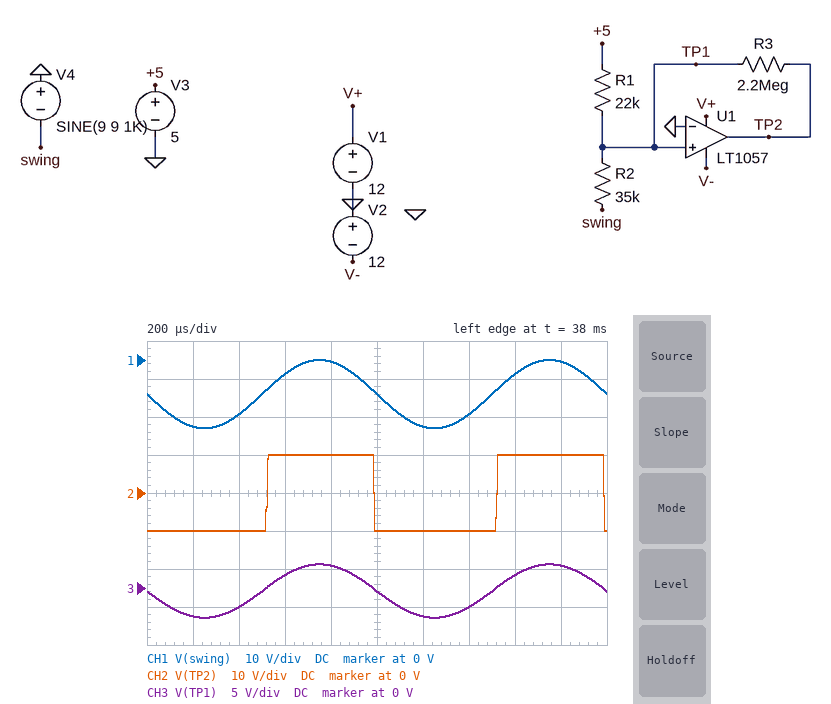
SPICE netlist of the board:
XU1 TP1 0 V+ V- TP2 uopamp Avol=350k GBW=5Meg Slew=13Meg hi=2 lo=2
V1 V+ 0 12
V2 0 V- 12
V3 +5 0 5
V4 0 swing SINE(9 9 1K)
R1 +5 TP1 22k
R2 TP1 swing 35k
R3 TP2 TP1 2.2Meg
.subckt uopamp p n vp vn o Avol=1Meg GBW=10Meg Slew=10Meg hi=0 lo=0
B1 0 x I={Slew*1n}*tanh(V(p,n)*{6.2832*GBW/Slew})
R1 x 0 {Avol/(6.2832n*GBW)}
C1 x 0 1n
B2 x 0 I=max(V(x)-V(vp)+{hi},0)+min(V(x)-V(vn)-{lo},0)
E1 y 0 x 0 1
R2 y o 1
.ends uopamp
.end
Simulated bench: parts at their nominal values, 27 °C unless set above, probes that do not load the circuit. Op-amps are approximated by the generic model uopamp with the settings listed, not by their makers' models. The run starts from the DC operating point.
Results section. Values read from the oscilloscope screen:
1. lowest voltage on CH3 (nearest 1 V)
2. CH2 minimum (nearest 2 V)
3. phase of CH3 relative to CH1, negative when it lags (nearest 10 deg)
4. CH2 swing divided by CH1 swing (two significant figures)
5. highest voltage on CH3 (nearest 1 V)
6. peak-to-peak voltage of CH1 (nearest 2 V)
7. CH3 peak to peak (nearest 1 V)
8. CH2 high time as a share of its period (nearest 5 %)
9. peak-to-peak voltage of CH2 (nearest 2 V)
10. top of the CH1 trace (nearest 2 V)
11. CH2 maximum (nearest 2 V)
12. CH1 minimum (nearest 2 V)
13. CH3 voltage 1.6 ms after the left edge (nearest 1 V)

-4 V
-10 V
0 deg
1.1
3 V
18 V
7 V
45 %
20 V
0 V
10 V
-18 V
2 V
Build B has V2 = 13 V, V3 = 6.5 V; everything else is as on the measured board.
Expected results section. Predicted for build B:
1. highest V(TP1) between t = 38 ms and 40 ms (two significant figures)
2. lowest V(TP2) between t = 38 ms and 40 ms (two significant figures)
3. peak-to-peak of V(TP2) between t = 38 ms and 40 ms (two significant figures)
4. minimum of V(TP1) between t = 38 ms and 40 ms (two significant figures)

4.0 V
-11 V
21 V
-3.0 V
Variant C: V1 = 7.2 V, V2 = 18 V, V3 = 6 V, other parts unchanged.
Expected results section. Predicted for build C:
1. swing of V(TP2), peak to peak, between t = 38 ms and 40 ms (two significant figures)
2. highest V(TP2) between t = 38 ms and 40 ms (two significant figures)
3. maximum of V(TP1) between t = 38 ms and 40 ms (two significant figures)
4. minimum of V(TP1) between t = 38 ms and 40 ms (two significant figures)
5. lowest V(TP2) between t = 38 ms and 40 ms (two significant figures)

21 V
5.2 V
3.7 V
-3.3 V
-16 V
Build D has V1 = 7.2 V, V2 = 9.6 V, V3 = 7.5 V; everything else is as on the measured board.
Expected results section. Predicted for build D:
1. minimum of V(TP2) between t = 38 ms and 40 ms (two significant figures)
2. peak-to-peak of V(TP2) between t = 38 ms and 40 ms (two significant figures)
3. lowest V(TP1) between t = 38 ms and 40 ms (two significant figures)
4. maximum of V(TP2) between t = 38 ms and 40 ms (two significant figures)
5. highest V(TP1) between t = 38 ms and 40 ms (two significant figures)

-7.6 V
13 V
-2.4 V
5.2 V
4.6 V
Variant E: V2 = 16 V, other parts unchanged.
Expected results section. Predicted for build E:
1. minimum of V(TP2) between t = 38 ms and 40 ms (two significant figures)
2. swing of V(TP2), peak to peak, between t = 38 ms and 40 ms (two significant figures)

-14 V
24 V
